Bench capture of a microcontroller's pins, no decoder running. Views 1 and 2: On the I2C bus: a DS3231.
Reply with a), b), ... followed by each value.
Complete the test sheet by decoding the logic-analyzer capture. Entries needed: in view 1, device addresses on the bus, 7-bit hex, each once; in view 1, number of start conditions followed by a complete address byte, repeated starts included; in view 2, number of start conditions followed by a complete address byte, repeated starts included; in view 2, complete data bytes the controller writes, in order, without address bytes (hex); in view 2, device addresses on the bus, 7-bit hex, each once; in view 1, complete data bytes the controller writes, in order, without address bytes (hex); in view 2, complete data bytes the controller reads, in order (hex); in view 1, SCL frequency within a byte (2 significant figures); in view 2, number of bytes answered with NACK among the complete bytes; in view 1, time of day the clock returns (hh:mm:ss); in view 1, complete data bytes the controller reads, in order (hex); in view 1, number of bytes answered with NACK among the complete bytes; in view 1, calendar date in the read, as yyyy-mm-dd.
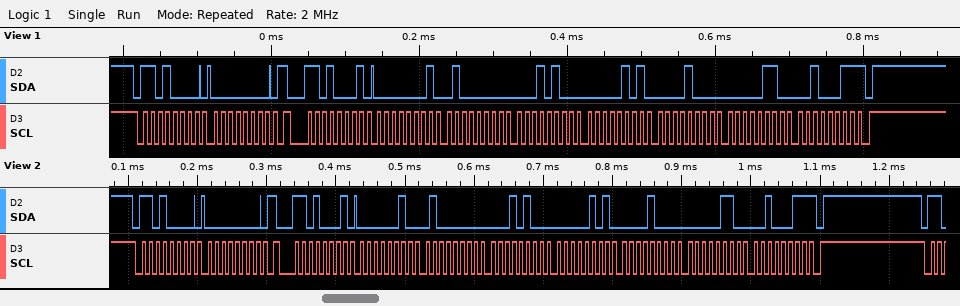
a) 0x68
b) 2
c) 2
d) 00
e) 0x68
f) 00
g) 02 40 14 05 08 06 23
h) 100 kHz
i) 1
j) 14:40:01
k) 01 40 14 05 08 06 23
l) 1
m) 2023-06-08
